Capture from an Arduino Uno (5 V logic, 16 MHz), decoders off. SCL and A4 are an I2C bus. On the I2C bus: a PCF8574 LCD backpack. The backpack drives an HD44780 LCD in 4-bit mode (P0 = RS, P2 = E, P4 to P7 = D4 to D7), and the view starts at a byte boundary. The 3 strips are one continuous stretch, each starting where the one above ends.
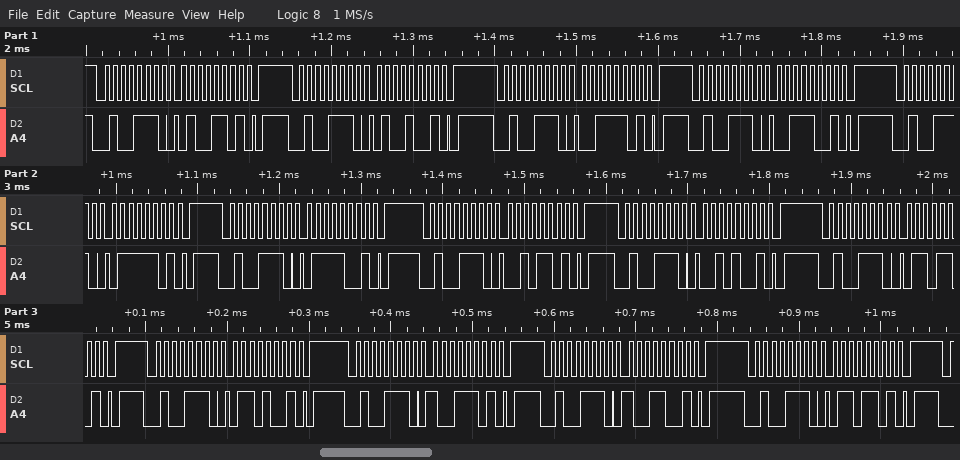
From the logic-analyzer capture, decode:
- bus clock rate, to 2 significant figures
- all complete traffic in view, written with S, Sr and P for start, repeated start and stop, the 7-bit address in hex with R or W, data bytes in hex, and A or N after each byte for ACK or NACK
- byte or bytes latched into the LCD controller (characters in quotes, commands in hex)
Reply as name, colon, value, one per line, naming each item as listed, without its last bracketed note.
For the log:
bus clock rate, to 2 significant figures: 100 kHz
all complete traffic in view, written with S, Sr and P for start, repeated start and stop, the 7-bit address in hex with R or W, data bytes in hex, and A or N after each byte for ACK or NACK: S 27W A 4D A P S 27W A 49 A P S 27W A 3D A P S 27W A 39 A P S 27W A 7D A P S 27W A 79 A P S 27W A 2D A P S 27W A 29 A P S 27W A 6D A P S 27W A 69 A P S 27W A 9D A P S 27W A 99 A P S 27W A 6D A P
byte or bytes latched into the LCD controller: 'C' 'r' 'i'
